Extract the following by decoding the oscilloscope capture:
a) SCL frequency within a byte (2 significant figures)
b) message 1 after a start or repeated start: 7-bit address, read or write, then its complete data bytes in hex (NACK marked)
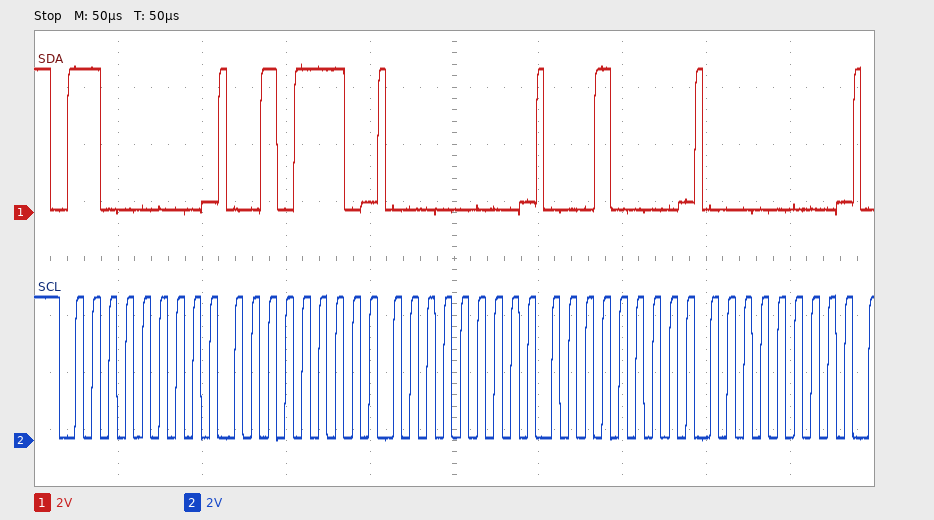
100 kHz
0x60 write: 2E 00 10 00
